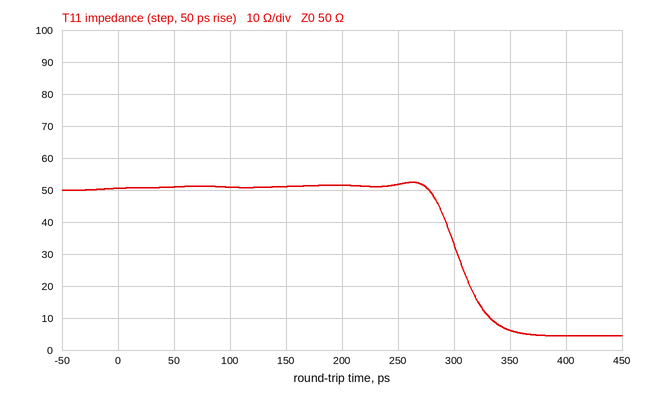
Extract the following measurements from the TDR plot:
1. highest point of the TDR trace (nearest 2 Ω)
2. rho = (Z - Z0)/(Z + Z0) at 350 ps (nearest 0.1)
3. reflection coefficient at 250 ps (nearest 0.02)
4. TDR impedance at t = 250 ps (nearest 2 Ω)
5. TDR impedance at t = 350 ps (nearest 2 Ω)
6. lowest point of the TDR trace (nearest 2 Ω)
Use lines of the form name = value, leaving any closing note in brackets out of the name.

highest point of the TDR trace = 52 Ω
rho = (Z - Z0)/(Z + Z0) at 350 ps = -0.8
reflection coefficient at 250 ps = +0.02
TDR impedance at t = 250 ps = 52 Ω
TDR impedance at t = 350 ps = 6 Ω
lowest point of the TDR trace = 4 Ω
